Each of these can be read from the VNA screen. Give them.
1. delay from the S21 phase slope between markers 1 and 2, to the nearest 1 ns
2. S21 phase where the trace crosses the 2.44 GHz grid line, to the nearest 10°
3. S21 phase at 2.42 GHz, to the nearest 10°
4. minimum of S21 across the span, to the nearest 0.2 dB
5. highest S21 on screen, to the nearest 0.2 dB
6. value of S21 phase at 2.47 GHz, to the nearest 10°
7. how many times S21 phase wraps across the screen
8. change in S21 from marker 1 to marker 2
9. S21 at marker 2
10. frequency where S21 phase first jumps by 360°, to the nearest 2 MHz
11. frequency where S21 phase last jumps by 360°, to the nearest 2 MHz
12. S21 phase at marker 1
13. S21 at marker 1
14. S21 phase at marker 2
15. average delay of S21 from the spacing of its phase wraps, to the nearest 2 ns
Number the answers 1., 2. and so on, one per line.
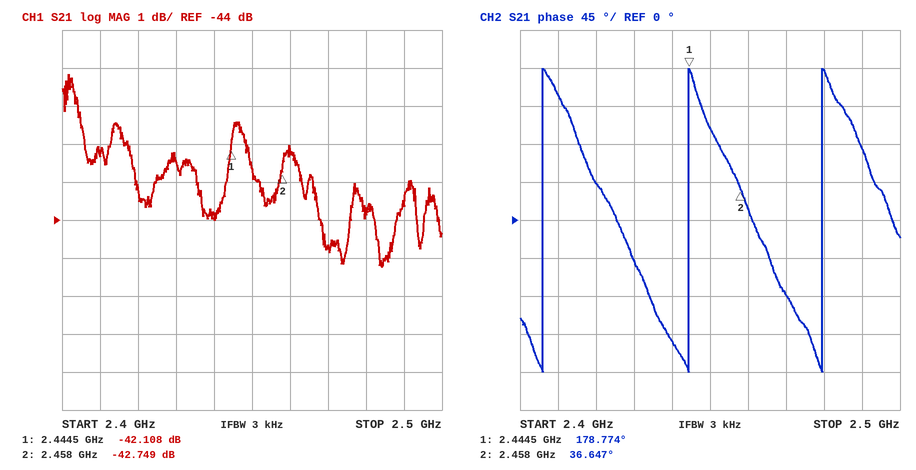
1. 29 ns
2. -140°
3. 40°
4. -45.2 dB
5. -40.2 dB
6. -90°
7. 3
8. -0.641 dB
9. -42.749 dB
10. 2.406 GHz
11. 2.480 GHz
12. 178.774°
13. -42.108 dB
14. 36.647°
15. 28 ns
